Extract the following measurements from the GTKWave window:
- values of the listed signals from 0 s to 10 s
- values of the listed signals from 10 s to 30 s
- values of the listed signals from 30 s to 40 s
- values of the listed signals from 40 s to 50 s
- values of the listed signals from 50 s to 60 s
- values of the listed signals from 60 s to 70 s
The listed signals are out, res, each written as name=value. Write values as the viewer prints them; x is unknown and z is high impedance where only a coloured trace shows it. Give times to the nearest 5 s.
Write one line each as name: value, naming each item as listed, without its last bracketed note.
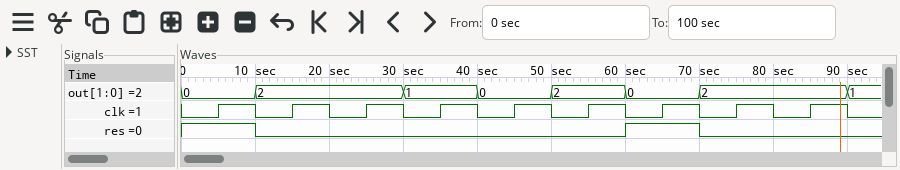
values of the listed signals from 0 s to 10 s: out=0, res=1
values of the listed signals from 10 s to 30 s: out=2, res=0
values of the listed signals from 30 s to 40 s: out=1, res=0
values of the listed signals from 40 s to 50 s: out=0, res=0
values of the listed signals from 50 s to 60 s: out=2, res=0
values of the listed signals from 60 s to 70 s: out=0, res=1
